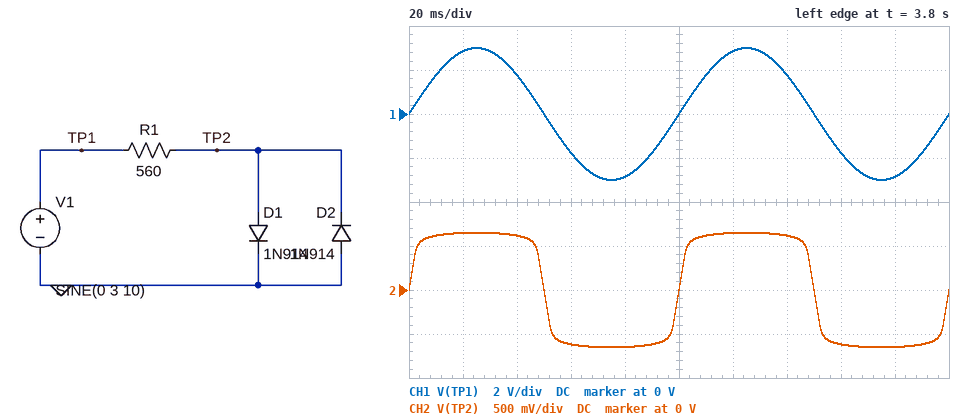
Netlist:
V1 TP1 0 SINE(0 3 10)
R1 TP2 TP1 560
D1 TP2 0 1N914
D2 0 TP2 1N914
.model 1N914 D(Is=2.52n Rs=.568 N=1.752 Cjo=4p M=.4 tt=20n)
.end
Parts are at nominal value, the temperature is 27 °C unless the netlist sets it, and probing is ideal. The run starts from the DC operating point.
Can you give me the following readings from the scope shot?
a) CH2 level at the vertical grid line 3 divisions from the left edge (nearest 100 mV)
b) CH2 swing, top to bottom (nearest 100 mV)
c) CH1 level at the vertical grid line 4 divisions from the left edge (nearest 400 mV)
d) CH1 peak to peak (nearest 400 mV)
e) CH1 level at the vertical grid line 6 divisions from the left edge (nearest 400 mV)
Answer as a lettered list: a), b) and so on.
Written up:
a) -600 mV
b) 1.3 V
c) -2.8 V
d) 6.0 V
e) 2.8 V
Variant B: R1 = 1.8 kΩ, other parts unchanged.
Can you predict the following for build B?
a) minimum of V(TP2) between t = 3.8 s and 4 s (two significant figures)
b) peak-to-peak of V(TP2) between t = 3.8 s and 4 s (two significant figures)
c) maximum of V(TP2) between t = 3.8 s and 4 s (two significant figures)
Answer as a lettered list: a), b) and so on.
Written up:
a) -600 mV
b) 1.2 V
c) 600 mV
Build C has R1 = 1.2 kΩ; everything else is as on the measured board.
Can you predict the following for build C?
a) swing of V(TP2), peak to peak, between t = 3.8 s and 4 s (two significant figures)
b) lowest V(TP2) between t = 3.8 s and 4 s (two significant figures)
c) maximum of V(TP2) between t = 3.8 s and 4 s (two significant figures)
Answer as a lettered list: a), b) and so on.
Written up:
a) 1.2 V
b) -620 mV
c) 620 mV
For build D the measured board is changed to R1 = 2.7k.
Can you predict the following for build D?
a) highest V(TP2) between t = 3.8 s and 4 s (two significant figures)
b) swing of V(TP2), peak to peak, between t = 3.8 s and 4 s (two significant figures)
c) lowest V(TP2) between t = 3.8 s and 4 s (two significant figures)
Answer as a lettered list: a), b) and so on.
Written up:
a) 580 mV
b) 1.2 V
c) -580 mV
